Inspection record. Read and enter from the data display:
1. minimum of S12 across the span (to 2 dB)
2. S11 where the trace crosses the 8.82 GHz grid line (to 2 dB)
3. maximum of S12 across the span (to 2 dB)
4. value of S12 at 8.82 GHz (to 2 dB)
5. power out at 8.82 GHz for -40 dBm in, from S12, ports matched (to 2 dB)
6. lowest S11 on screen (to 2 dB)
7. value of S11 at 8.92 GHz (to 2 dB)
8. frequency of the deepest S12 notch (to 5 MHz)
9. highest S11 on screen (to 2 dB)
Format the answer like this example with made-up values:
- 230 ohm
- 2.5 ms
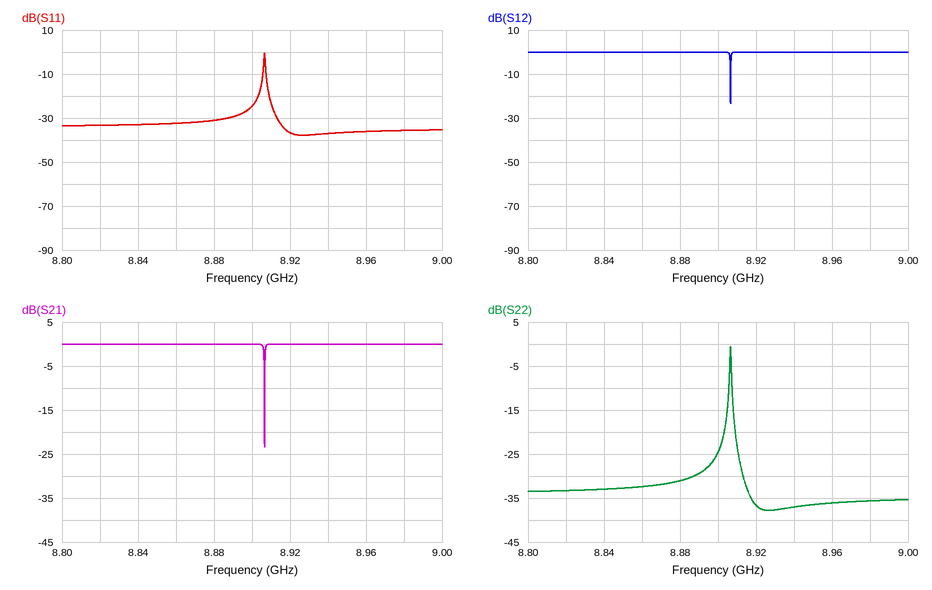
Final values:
- -24 dB
- -34 dB
- 0 dB
- 0 dB
- -40 dBm
- -38 dB
- -36 dB
- 8.905 GHz
- 0 dB
